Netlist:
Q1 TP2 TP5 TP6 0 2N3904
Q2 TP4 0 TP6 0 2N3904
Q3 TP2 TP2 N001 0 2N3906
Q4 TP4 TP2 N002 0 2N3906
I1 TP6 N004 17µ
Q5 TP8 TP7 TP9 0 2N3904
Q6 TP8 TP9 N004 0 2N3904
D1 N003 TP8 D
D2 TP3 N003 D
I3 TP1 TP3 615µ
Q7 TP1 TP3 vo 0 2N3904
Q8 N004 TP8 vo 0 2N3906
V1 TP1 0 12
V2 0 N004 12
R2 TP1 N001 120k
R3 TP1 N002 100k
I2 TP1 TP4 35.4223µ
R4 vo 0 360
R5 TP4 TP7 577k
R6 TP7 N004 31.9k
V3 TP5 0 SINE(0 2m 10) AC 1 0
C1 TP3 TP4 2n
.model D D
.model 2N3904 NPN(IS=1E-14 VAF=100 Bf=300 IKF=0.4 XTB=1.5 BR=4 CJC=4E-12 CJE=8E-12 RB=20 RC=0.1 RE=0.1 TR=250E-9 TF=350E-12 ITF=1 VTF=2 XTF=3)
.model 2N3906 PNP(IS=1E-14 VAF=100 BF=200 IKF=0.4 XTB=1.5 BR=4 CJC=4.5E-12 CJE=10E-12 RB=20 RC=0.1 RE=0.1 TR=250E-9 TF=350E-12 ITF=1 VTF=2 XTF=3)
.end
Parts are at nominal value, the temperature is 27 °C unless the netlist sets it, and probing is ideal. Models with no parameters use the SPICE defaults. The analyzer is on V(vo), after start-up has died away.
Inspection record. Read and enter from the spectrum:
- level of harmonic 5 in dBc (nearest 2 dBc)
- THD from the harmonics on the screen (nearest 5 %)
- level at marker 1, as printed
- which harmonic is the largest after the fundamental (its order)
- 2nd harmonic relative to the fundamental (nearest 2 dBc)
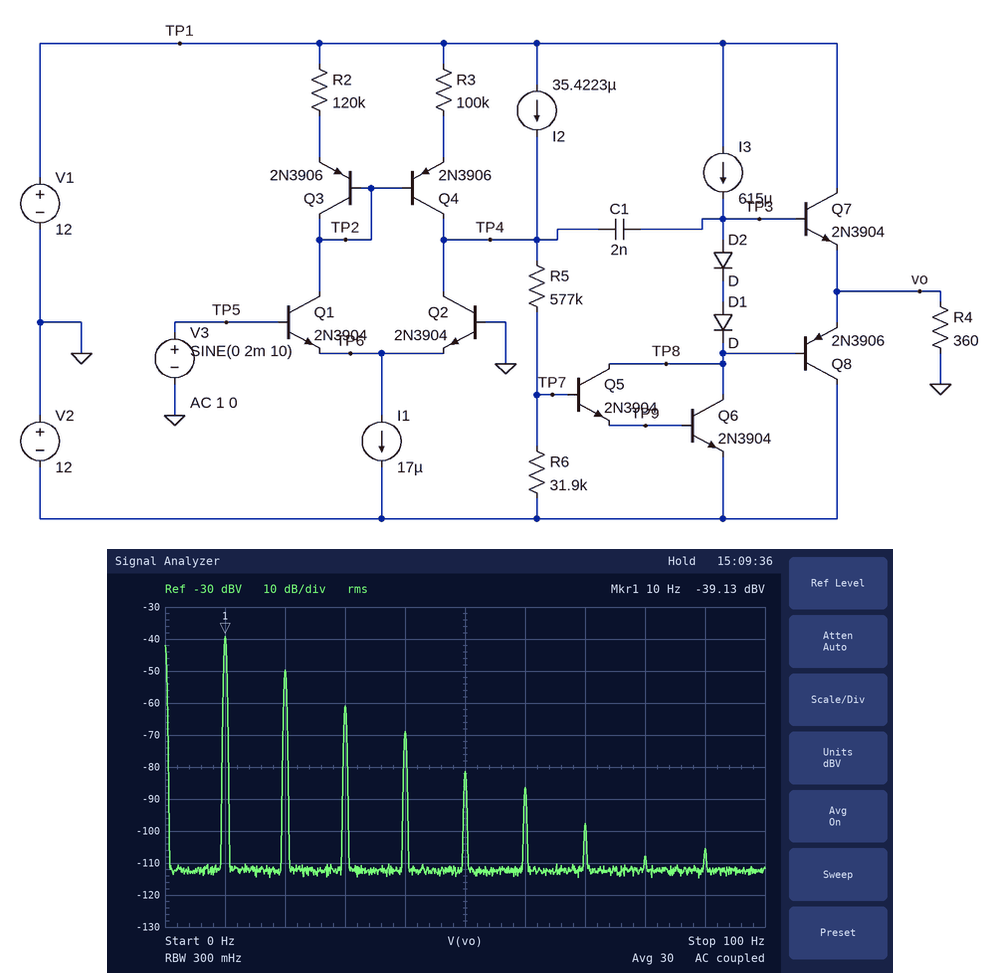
-42 dBc
30 %
-39.13 dBV
2
-10 dBc
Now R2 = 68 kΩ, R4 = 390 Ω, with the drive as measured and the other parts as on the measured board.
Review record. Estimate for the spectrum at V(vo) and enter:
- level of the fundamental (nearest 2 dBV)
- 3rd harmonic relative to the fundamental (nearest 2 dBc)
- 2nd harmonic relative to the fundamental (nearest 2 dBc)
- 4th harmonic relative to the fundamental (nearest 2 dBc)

-52 dBV
-38 dBc
-18 dBc
-58 dBc
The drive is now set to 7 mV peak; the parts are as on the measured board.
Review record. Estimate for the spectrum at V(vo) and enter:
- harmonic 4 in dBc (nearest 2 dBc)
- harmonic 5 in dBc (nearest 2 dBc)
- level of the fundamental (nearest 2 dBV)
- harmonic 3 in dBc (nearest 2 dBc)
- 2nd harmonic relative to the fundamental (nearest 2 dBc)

-22 dBc
-28 dBc
12 dBV
-20 dBc
-6 dBc
